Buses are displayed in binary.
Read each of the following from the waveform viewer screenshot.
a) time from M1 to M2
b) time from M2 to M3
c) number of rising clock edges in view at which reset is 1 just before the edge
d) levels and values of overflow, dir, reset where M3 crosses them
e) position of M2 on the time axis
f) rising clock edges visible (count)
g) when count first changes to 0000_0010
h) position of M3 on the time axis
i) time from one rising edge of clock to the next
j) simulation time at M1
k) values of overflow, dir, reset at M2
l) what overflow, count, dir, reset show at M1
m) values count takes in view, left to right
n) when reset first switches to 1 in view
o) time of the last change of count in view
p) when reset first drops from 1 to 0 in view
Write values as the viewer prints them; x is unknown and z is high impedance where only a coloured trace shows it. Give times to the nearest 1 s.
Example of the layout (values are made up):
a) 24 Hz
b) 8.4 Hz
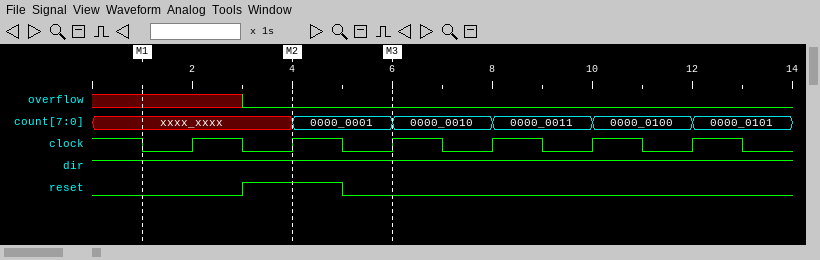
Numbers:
a) 3 s
b) 2 s
c) 1
d) overflow=0, dir=1, reset=0
e) 4 s
f) 6
g) 6 s
h) 6 s
i) 2 s
j) 1 s
k) overflow=0, dir=1, reset=1
l) overflow=x, count=xxxx_xxxx, dir=1, reset=0
m) xxxx_xxxx, 0000_0001, 0000_0010, 0000_0011, 0000_0100, 0000_0101
n) 3 s
o) 12 s
p) 5 s
